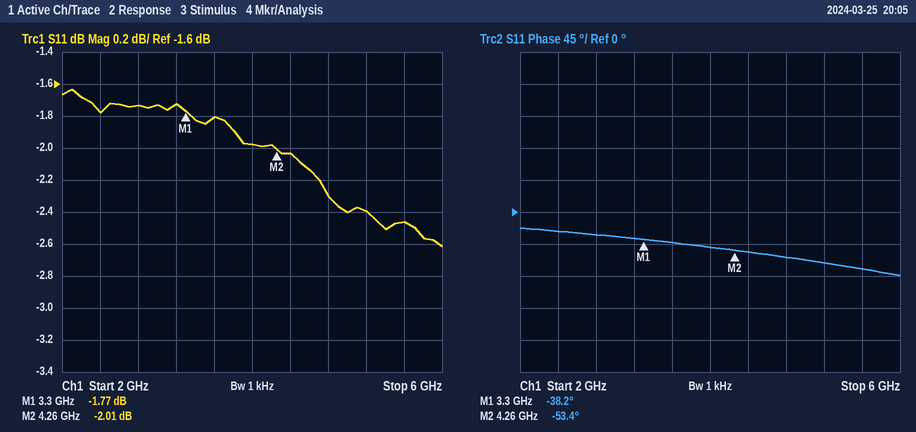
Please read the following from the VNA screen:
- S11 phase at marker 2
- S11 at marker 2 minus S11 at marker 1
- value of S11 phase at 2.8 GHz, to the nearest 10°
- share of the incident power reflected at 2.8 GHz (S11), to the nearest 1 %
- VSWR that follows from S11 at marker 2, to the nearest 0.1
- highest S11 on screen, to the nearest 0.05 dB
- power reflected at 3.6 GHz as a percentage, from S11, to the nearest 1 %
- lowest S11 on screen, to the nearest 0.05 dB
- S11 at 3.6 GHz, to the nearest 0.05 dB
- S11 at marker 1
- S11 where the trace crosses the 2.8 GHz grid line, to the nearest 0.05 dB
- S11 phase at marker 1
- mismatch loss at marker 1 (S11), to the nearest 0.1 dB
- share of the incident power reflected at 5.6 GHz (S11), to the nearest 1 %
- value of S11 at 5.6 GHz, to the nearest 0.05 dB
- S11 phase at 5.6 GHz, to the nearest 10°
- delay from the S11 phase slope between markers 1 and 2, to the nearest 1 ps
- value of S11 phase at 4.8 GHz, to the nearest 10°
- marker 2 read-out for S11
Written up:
-53.4°
-0.24 dB
-30°
67 %
8.7
-1.65 dB
66 %
-2.60 dB
-1.80 dB
-1.77 dB
-1.75 dB
-38.2°
4.8 dB
57 %
-2.45 dB
-80°
44 ps
-60°
-2.01 dB
